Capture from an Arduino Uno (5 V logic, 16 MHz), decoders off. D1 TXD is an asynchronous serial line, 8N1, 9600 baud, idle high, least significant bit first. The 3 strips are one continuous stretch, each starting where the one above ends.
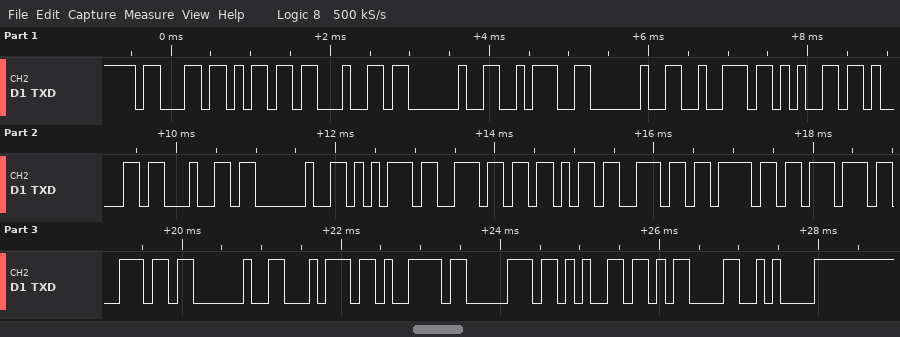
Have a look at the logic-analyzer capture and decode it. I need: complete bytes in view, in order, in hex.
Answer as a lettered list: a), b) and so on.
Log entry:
a) 63 6D 64 20 3A 20 72 65 61 64 20 75 6E 6B 6E 6F 77 6E 20 74 79 70 65 0D 0A
